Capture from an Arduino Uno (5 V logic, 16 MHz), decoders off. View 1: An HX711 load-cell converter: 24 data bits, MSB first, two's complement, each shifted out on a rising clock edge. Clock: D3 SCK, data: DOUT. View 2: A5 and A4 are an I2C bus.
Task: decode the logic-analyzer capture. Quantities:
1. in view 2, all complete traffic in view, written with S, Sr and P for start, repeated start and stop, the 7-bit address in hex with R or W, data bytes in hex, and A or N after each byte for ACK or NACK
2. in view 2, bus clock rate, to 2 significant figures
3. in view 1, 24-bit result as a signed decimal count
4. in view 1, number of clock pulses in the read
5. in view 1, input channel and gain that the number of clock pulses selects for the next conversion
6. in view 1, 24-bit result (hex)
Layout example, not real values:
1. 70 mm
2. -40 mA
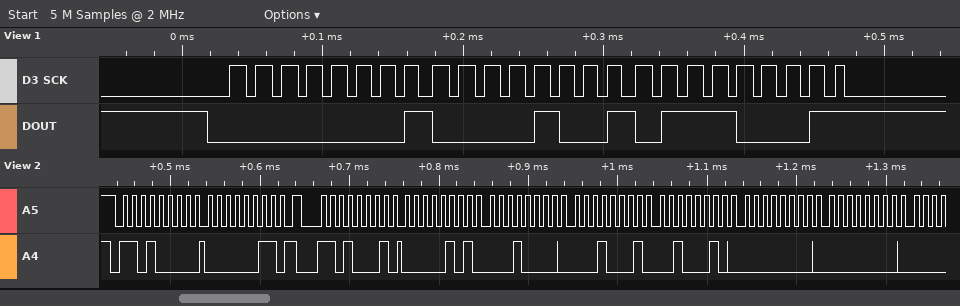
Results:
1. S 68W A 03 A Sr 68R A 05 A 10 A 11 A 22 A 00 A 00 A
2. 100 kHz
3. 67953
4. 25
5. channel A, gain 128
6. 0x010971
